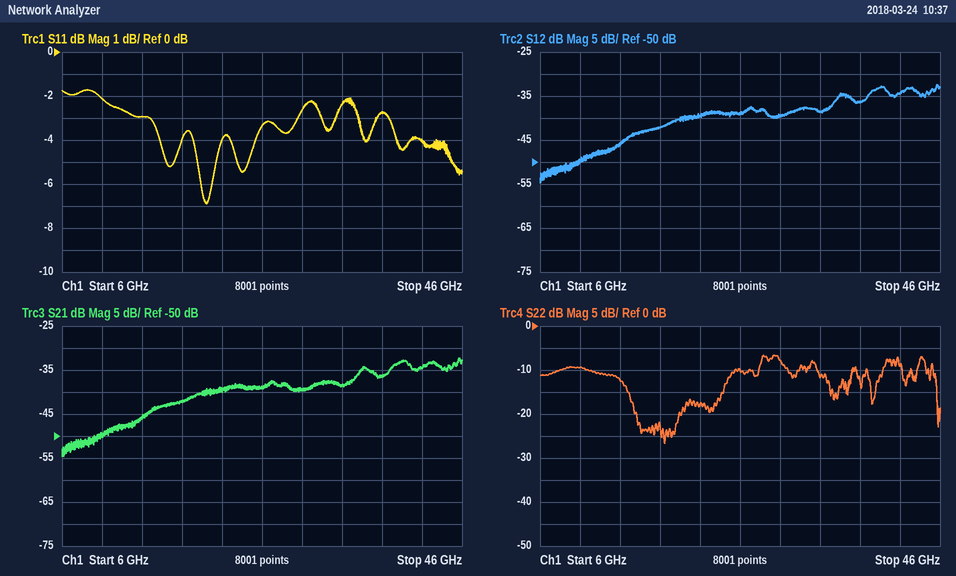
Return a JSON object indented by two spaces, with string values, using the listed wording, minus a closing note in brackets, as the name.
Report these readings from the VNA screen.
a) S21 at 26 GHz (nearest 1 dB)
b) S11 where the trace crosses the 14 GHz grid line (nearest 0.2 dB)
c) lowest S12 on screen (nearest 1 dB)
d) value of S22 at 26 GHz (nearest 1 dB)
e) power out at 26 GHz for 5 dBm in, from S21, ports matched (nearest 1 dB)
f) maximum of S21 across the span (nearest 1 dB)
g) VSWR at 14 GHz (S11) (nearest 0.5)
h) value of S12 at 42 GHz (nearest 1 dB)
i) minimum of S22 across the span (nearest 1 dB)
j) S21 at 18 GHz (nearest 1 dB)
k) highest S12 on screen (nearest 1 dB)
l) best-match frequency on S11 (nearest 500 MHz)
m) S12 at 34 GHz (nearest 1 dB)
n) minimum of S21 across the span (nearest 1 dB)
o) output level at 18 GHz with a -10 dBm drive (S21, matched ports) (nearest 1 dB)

{
  "S21 at 26 GHz": "-39 dB",
  "S11 where the trace crosses the 14 GHz grid line": "-3.0 dB",
  "lowest S12 on screen": "-55 dB",
  "value of S22 at 26 GHz": "-10 dB",
  "power out at 26 GHz for 5 dBm in, from S21, ports matched": "-34 dBm",
  "maximum of S21 across the span": "-32 dB",
  "VSWR at 14 GHz (S11)": "6.0",
  "value of S12 at 42 GHz": "-34 dB",
  "minimum of S22 across the span": "-27 dB",
  "S21 at 18 GHz": "-42 dB",
  "highest S12 on screen": "-32 dB",
  "best-match frequency on S11": "20.5 GHz",
  "S12 at 34 GHz": "-39 dB",
  "minimum of S21 across the span": "-55 dB",
  "output level at 18 GHz with a -10 dBm drive (S21, matched ports)": "-52 dBm"
}
